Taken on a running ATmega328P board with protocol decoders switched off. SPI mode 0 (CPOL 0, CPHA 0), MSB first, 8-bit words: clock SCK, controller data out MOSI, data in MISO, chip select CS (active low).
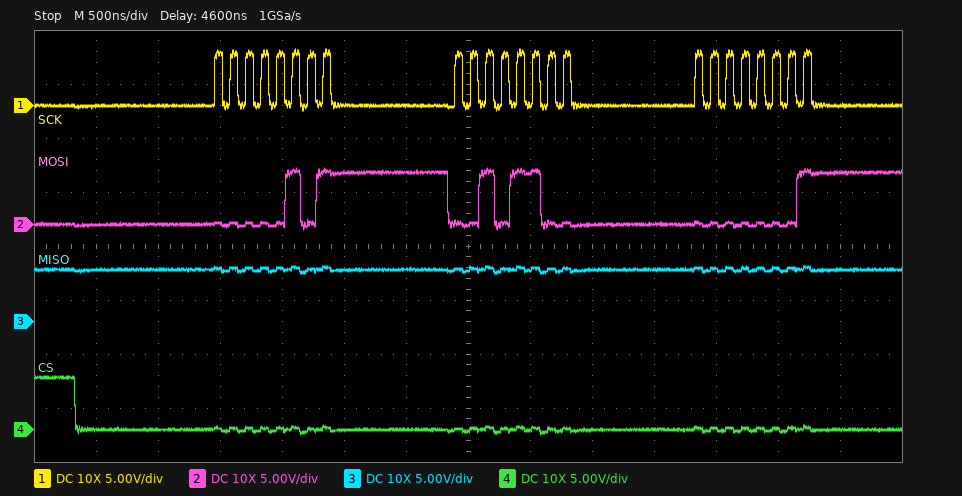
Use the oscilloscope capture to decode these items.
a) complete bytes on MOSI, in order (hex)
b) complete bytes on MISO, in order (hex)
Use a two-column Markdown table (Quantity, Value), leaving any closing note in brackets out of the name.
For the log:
| Quantity | Value |
|---|---|
| complete bytes on MOSI, in order | 0x05 0x2C 0x01 |
| complete bytes on MISO, in order | 0xFF 0xFF 0xFF |
